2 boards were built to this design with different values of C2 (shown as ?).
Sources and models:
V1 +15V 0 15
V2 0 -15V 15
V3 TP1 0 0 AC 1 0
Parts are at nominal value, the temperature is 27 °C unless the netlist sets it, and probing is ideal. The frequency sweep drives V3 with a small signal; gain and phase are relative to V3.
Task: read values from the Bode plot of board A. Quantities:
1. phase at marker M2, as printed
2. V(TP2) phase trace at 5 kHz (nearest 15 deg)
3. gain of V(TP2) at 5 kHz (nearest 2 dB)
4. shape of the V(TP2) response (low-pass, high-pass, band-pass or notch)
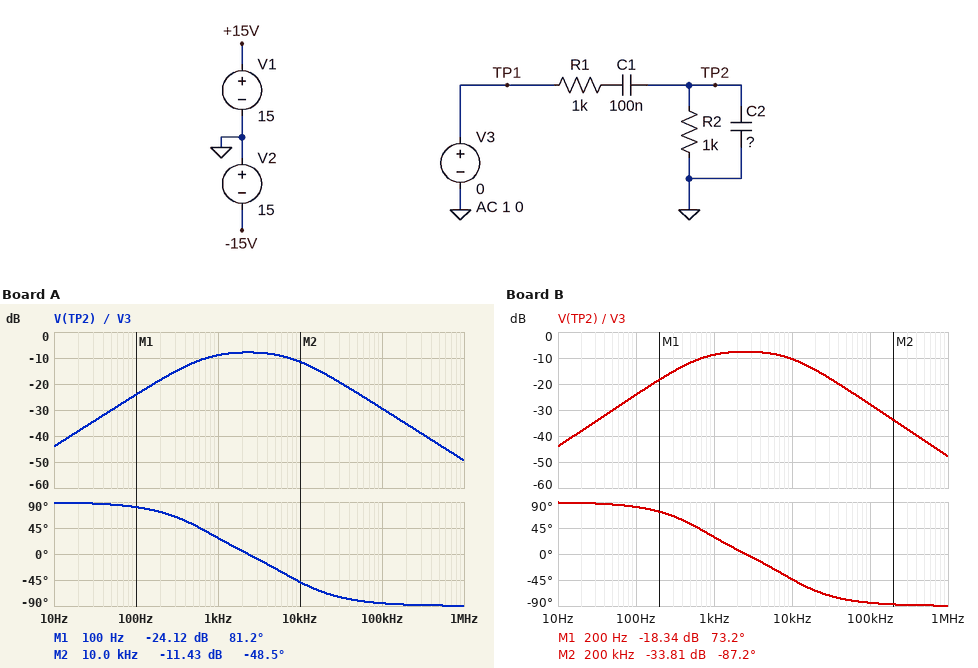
-48.5 deg
-30 deg
-8 dB
band-pass
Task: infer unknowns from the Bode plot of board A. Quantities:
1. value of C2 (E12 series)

47 nF
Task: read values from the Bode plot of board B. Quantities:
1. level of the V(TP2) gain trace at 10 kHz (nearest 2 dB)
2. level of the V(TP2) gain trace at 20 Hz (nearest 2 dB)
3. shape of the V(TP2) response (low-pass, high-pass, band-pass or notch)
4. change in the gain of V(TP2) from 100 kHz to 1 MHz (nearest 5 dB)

-10 dB
-38 dB
band-pass
-20 dB
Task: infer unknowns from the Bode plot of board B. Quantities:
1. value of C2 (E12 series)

39 nF
